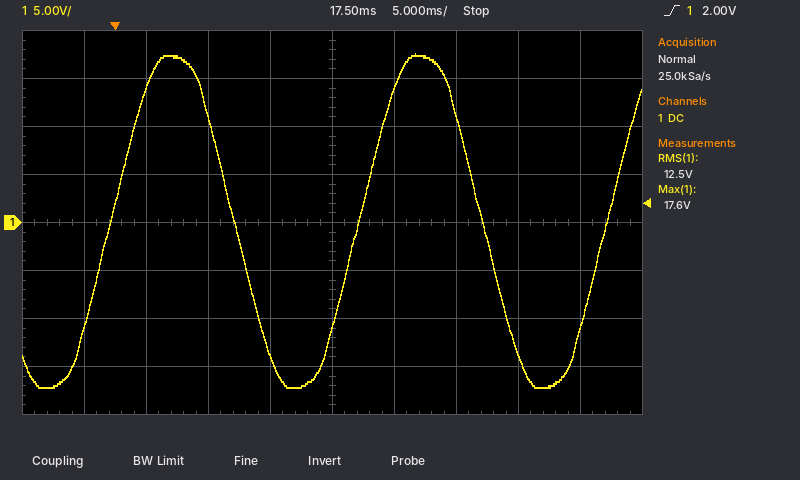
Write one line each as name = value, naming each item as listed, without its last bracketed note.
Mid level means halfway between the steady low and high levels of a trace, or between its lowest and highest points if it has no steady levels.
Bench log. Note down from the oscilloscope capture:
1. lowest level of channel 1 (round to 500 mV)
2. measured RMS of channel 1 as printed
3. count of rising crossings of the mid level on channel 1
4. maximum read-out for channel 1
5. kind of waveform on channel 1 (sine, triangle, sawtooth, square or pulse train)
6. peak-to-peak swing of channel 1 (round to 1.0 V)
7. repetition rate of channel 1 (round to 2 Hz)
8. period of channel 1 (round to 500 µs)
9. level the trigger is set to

lowest level of channel 1 = -17.0 V
measured RMS of channel 1 as printed = 12.5 V
count of rising crossings of the mid level on channel 1 = 3
maximum read-out for channel 1 = 17.6 V
kind of waveform on channel 1 = sine
peak-to-peak swing of channel 1 = 35.0 V
repetition rate of channel 1 = 50 Hz
period of channel 1 = 20.0 ms
level the trigger is set to = 2.00 V
